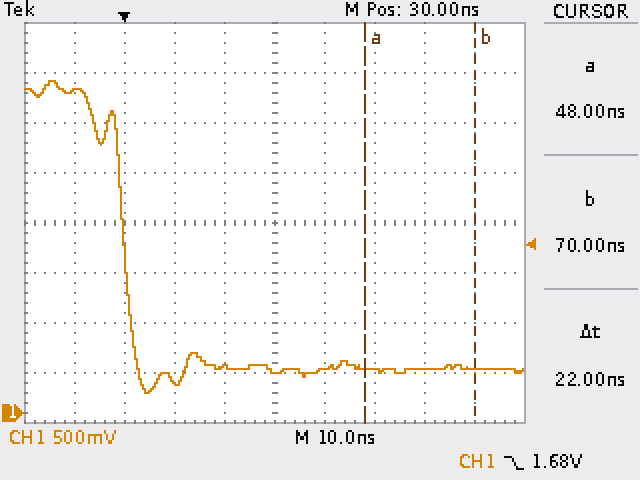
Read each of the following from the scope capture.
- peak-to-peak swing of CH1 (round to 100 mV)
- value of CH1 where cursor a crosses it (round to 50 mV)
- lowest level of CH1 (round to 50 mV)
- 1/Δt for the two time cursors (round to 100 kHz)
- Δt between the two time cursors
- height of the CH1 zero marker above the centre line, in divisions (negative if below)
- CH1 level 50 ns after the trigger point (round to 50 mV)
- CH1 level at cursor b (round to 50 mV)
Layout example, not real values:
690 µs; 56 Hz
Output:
3.10 V; 450 mV; 200 mV; 45.5 MHz; 22 ns; -3.8 div; 450 mV; 450 mV
